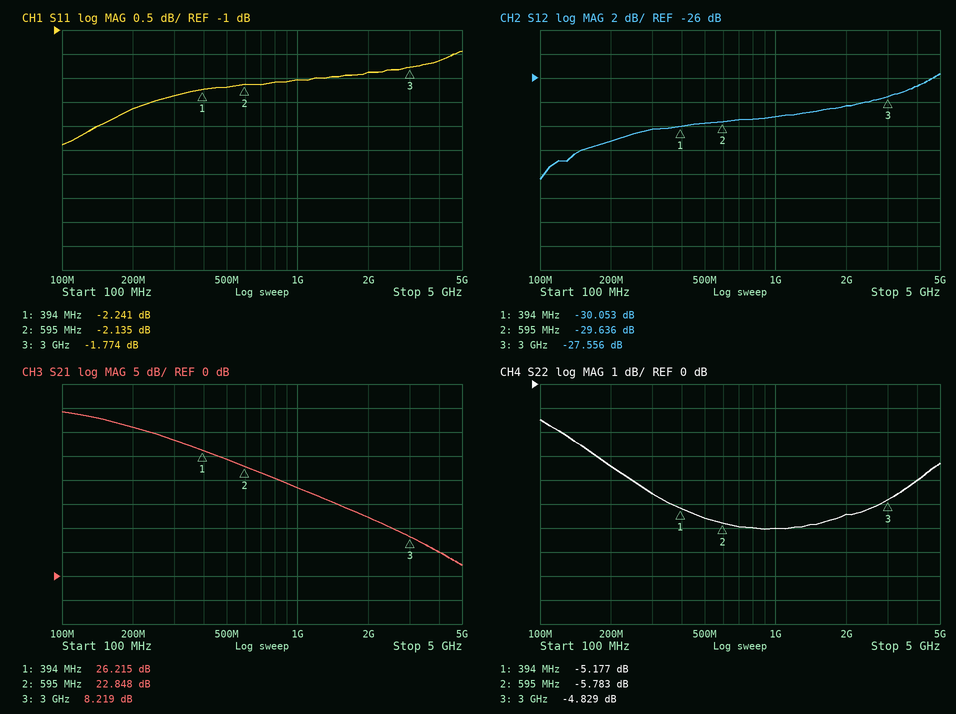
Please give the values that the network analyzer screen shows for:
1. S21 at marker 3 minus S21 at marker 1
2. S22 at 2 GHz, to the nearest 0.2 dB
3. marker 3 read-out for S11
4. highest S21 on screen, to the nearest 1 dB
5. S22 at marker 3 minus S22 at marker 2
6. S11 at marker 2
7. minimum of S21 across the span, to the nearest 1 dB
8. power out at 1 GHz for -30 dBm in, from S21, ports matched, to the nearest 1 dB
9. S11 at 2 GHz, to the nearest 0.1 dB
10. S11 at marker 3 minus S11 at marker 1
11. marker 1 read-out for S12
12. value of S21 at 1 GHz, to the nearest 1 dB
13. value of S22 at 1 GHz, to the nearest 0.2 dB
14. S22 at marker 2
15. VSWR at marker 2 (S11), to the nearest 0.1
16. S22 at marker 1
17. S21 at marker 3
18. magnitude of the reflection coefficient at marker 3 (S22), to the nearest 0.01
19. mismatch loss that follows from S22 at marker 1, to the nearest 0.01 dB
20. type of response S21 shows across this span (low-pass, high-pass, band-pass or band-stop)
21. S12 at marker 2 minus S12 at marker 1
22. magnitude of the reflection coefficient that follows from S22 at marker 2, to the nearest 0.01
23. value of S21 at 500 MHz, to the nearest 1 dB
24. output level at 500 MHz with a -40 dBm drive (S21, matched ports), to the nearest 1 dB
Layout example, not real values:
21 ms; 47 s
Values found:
-17.996 dB; -5.4 dB; -1.774 dB; 34 dB; 0.954 dB; -2.135 dB; 2 dB; -12 dBm; -1.9 dB; 0.467 dB; -30.053 dB; 18 dB; -6.0 dB; -5.783 dB; 8.2; -5.177 dB; 8.219 dB; 0.57; 1.57 dB; low-pass; 0.417 dB; 0.51; 24 dB; -16 dBm
